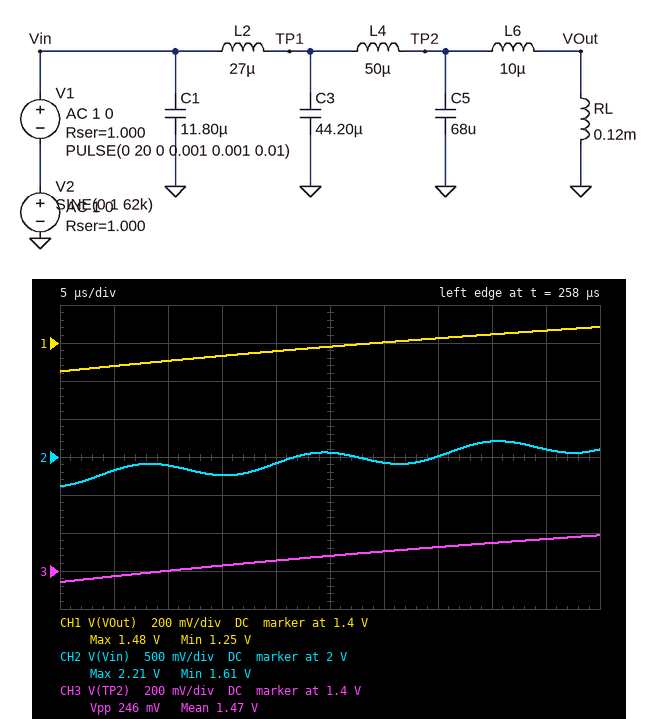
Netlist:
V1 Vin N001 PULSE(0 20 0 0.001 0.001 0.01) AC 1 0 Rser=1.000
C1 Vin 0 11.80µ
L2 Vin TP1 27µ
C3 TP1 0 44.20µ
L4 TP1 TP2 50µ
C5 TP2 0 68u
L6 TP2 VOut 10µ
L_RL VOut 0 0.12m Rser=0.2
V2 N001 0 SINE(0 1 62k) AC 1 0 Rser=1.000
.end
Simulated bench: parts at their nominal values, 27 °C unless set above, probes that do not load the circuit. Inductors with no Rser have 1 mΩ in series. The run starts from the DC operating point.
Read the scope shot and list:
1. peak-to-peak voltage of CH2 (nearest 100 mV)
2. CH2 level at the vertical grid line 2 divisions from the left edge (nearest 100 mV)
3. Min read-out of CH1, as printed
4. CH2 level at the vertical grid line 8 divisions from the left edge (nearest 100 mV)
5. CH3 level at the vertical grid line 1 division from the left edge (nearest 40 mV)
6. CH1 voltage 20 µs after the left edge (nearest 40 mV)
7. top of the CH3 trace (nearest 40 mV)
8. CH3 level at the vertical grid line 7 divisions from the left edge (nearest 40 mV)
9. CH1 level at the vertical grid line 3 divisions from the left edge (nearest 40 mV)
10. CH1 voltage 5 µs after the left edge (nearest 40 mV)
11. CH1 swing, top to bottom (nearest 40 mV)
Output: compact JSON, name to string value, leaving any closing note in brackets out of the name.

{"peak-to-peak voltage of CH2": "600 mV", "CH2 level at the vertical grid line 2 divisions from the left edge": "1.9 V", "Min read-out of CH1, as printed": "1.25 V", "CH2 level at the vertical grid line 8 divisions from the left edge": "2.2 V", "CH3 level at the vertical grid line 1 division from the left edge": "1.36 V", "CH1 voltage 20 µs after the left edge": "1.36 V", "top of the CH3 trace": "1.60 V", "CH3 level at the vertical grid line 7 divisions from the left edge": "1.52 V", "CH1 level at the vertical grid line 3 divisions from the left edge": "1.32 V", "CH1 voltage 5 µs after the left edge": "1.28 V", "CH1 swing, top to bottom": "240 mV"}
